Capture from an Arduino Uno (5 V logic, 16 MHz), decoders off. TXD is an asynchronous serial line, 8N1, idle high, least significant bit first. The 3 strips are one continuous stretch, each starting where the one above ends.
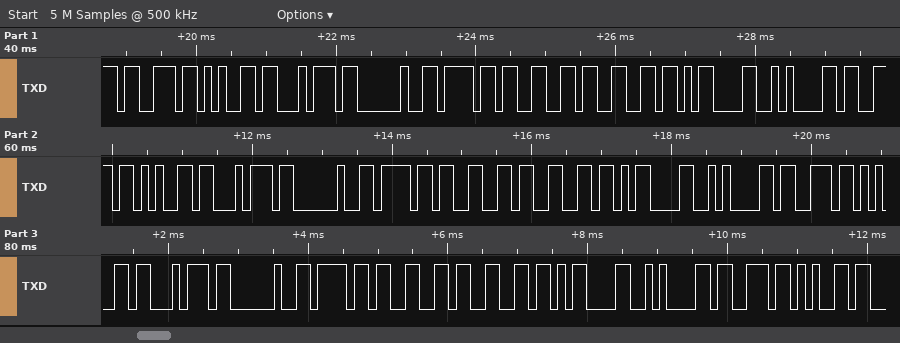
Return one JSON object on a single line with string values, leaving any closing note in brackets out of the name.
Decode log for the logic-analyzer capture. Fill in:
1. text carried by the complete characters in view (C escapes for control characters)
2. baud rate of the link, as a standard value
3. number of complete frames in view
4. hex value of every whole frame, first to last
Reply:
{"text carried by the complete characters in view": "\"set off\\r\\nset off\\r\\nset off\\r\\nse\"", "baud rate of the link, as a standard value": "9600 baud", "number of complete frames in view": "29", "hex value of every whole frame, first to last": "73 65 74 20 6F 66 66 0D 0A 73 65 74 20 6F 66 66 0D 0A 73 65 74 20 6F 66 66 0D 0A 73 65"}
